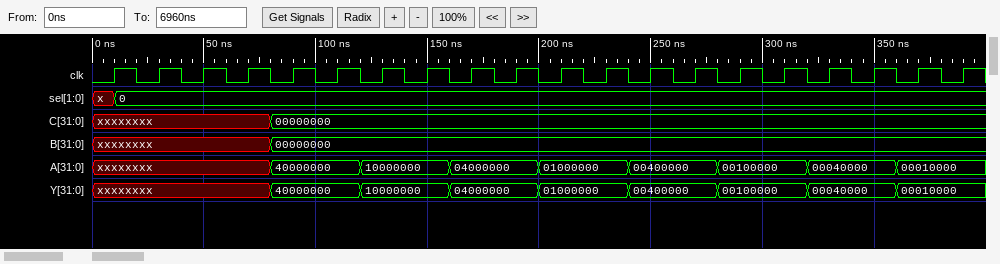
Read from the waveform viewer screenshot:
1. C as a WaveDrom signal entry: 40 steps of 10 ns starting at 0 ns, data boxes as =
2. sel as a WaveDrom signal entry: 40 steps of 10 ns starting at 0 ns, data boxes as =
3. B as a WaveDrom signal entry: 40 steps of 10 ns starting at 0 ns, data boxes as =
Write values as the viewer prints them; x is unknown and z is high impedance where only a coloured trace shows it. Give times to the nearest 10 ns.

{name: 'C', wave: 'x.......=...............................', data: '00000000'}
{name: 'sel', wave: 'x=......................................', data: '0'}
{name: 'B', wave: 'x.......=...............................', data: '00000000'}
